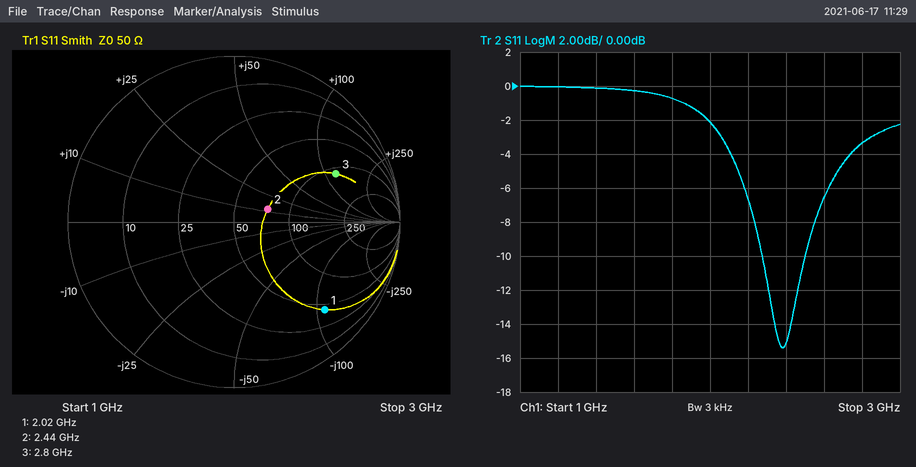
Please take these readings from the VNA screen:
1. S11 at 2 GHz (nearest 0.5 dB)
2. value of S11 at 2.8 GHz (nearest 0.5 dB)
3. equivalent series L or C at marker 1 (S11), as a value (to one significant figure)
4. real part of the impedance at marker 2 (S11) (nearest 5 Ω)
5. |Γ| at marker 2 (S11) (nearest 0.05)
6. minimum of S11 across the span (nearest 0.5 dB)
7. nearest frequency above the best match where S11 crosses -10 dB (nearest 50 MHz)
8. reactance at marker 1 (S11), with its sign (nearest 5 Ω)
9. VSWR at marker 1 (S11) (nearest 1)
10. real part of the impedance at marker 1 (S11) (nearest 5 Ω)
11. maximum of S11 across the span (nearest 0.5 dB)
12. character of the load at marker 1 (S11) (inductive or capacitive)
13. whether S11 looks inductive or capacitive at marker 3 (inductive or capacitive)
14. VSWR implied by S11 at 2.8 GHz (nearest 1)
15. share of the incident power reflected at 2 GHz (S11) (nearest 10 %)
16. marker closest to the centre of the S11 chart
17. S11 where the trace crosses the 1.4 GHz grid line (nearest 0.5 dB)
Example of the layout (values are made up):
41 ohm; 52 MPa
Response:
-2.0 dB; -3.5 dB; 700 fF; 75 Ω; 0.20; -15.5 dB; 2.50 GHz; -110 Ω; 7; 45 Ω; 0.0 dB; capacitive; inductive; 5; 60 %; marker 2; 0.0 dB
